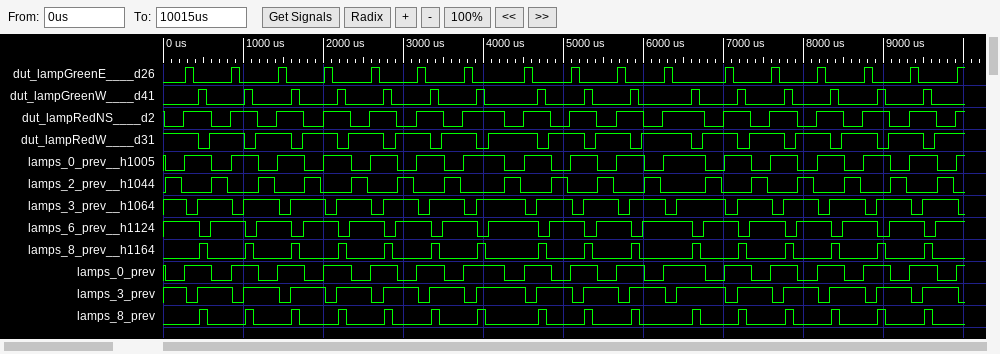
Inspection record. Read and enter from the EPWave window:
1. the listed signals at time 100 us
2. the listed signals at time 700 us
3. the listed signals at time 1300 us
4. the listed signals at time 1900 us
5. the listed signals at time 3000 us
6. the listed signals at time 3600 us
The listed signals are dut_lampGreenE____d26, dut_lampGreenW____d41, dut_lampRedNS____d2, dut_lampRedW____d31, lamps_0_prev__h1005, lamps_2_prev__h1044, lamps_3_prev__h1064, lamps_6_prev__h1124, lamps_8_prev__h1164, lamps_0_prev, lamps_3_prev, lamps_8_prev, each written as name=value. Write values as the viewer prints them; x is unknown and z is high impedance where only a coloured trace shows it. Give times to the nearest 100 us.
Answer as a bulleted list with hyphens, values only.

- dut_lampGreenE____d26=0, dut_lampGreenW____d41=0, dut_lampRedNS____d2=0, dut_lampRedW____d31=1, lamps_0_prev__h1005=0, lamps_2_prev__h1044=1, lamps_3_prev__h1064=1, lamps_6_prev__h1124=1, lamps_8_prev__h1164=0, lamps_0_prev=0, lamps_3_prev=1, lamps_8_prev=0
- dut_lampGreenE____d26=0, dut_lampGreenW____d41=0, dut_lampRedNS____d2=0, dut_lampRedW____d31=1, lamps_0_prev__h1005=0, lamps_2_prev__h1044=1, lamps_3_prev__h1064=1, lamps_6_prev__h1124=1, lamps_8_prev__h1164=0, lamps_0_prev=0, lamps_3_prev=1, lamps_8_prev=0
- dut_lampGreenE____d26=0, dut_lampGreenW____d41=0, dut_lampRedNS____d2=0, dut_lampRedW____d31=1, lamps_0_prev__h1005=0, lamps_2_prev__h1044=1, lamps_3_prev__h1064=1, lamps_6_prev__h1124=1, lamps_8_prev__h1164=0, lamps_0_prev=0, lamps_3_prev=1, lamps_8_prev=0
- dut_lampGreenE____d26=0, dut_lampGreenW____d41=0, dut_lampRedNS____d2=0, dut_lampRedW____d31=1, lamps_0_prev__h1005=0, lamps_2_prev__h1044=1, lamps_3_prev__h1064=1, lamps_6_prev__h1124=1, lamps_8_prev__h1164=0, lamps_0_prev=0, lamps_3_prev=1, lamps_8_prev=0
- dut_lampGreenE____d26=0, dut_lampGreenW____d41=0, dut_lampRedNS____d2=0, dut_lampRedW____d31=1, lamps_0_prev__h1005=0, lamps_2_prev__h1044=1, lamps_3_prev__h1064=1, lamps_6_prev__h1124=1, lamps_8_prev__h1164=0, lamps_0_prev=0, lamps_3_prev=1, lamps_8_prev=0
- dut_lampGreenE____d26=0, dut_lampGreenW____d41=0, dut_lampRedNS____d2=0, dut_lampRedW____d31=1, lamps_0_prev__h1005=0, lamps_2_prev__h1044=1, lamps_3_prev__h1064=1, lamps_6_prev__h1124=1, lamps_8_prev__h1164=0, lamps_0_prev=0, lamps_3_prev=1, lamps_8_prev=0
